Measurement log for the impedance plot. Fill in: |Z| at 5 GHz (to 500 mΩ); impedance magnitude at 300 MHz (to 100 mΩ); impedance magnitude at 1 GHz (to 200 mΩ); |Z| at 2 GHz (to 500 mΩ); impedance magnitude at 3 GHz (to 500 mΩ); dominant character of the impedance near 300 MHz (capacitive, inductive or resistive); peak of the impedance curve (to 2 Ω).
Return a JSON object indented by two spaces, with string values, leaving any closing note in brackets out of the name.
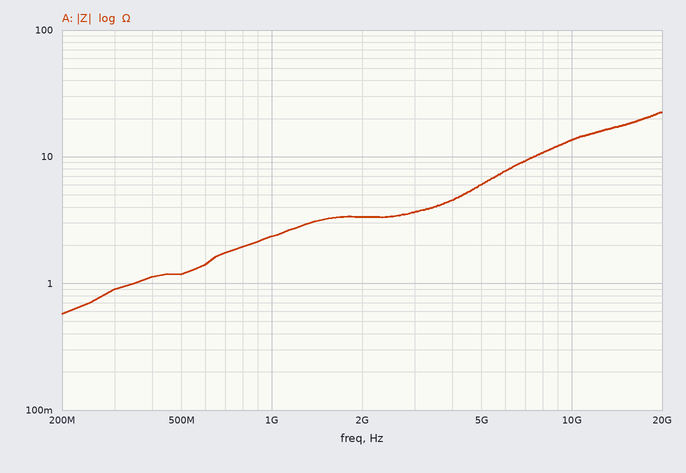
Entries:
{
  "|Z| at 5 GHz": "6.0 Ω",
  "impedance magnitude at 300 MHz": "900 mΩ",
  "impedance magnitude at 1 GHz": "2.4 Ω",
  "|Z| at 2 GHz": "3.5 Ω",
  "impedance magnitude at 3 GHz": "3.5 Ω",
  "dominant character of the impedance near 300 MHz": "inductive",
  "peak of the impedance curve": "22 Ω"
}
